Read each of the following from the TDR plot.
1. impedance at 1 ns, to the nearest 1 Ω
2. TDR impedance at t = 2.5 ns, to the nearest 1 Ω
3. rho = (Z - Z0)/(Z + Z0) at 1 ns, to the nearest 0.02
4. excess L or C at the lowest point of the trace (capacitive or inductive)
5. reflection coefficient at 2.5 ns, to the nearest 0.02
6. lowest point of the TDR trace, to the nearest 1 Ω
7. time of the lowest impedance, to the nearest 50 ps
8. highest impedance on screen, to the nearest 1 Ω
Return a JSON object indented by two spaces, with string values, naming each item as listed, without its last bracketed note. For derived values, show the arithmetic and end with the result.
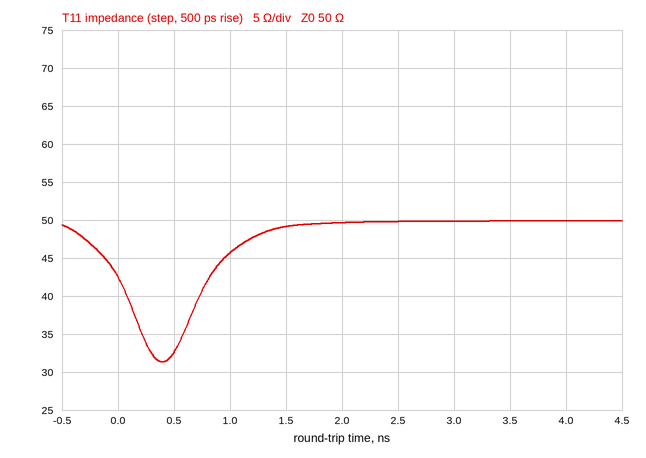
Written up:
{
  "impedance at 1 ns, to the nearest 1 Ω": "46 Ω",
  "TDR impedance at t = 2.5 ns, to the nearest 1 Ω": "50 Ω",
  "rho = (Z - Z0)/(Z + Z0) at 1 ns, to the nearest 0.02": "(46 − 50)/(46 + 50) ≈ -0.04",
  "excess L or C at the lowest point of the trace": "capacitive",
  "reflection coefficient at 2.5 ns, to the nearest 0.02": "(50 − 50)/(50 + 50) ≈ 0.00",
  "lowest point of the TDR trace, to the nearest 1 Ω": "31 Ω",
  "time of the lowest impedance, to the nearest 50 ps": "400 ps",
  "highest impedance on screen, to the nearest 1 Ω": "50 Ω"
}
